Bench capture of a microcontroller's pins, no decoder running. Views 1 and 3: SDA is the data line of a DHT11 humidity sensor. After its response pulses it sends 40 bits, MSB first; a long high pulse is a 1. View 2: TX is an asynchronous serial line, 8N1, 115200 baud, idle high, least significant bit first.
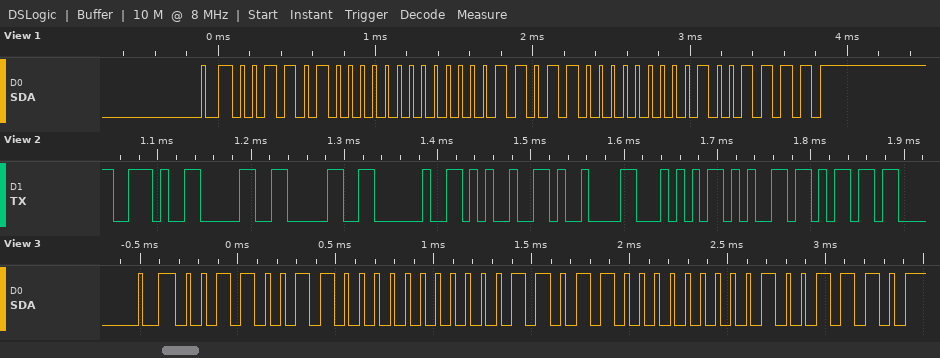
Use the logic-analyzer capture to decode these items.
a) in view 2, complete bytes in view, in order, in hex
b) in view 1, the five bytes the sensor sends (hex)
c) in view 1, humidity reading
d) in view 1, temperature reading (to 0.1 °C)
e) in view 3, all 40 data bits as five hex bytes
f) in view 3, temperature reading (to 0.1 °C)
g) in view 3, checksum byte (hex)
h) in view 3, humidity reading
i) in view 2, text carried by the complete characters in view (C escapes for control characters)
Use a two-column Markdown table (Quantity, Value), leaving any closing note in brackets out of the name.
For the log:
| Quantity | Value |
|---|---|
| in view 2, complete bytes in view, in order, in hex | 2E 30 30 20 25 09 54 65 6D |
| in view 1, the five bytes the sensor sends | 34 00 1B 00 4F |
| in view 1, humidity reading | 52 % |
| in view 1, temperature reading | 27.0 °C |
| in view 3, all 40 data bits as five hex bytes | 33 00 1B 00 4E |
| in view 3, temperature reading | 27.0 °C |
| in view 3, checksum byte | 0x4E |
| in view 3, humidity reading | 51 % |
| in view 2, text carried by the complete characters in view | ".00 %\tTem" |
